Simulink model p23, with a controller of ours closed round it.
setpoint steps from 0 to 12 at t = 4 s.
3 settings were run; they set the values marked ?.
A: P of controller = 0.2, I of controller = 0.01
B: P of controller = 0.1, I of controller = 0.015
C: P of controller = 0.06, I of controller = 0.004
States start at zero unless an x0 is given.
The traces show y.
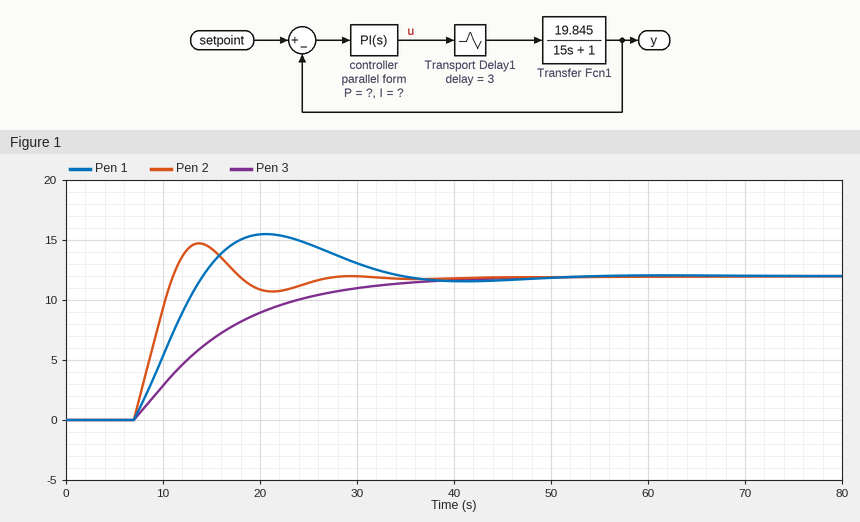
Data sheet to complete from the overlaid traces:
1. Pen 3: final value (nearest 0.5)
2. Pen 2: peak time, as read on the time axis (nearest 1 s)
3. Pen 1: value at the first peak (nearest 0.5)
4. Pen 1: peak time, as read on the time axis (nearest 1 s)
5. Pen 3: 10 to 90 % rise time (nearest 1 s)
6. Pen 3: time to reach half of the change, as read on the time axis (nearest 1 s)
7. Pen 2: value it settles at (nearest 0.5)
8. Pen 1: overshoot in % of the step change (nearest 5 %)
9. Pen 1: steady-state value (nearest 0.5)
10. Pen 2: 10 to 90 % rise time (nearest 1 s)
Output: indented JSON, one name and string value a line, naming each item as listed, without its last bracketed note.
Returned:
{
  "Pen 3: final value": "12.0",
  "Pen 2: peak time, as read on the time axis": "14 s",
  "Pen 1: value at the first peak": "15.5",
  "Pen 1: peak time, as read on the time axis": "21 s",
  "Pen 3: 10 to 90 % rise time": "20 s",
  "Pen 3: time to reach half of the change, as read on the time axis": "14 s",
  "Pen 2: value it settles at": "12.0",
  "Pen 1: overshoot in % of the step change": "30 %",
  "Pen 1: steady-state value": "12.0",
  "Pen 2: 10 to 90 % rise time": "3 s"
}
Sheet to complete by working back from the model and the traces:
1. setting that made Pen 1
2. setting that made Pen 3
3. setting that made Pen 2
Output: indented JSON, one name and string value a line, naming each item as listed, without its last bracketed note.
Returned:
{
  "setting that made Pen 1": "B",
  "setting that made Pen 3": "C",
  "setting that made Pen 2": "A"
}
